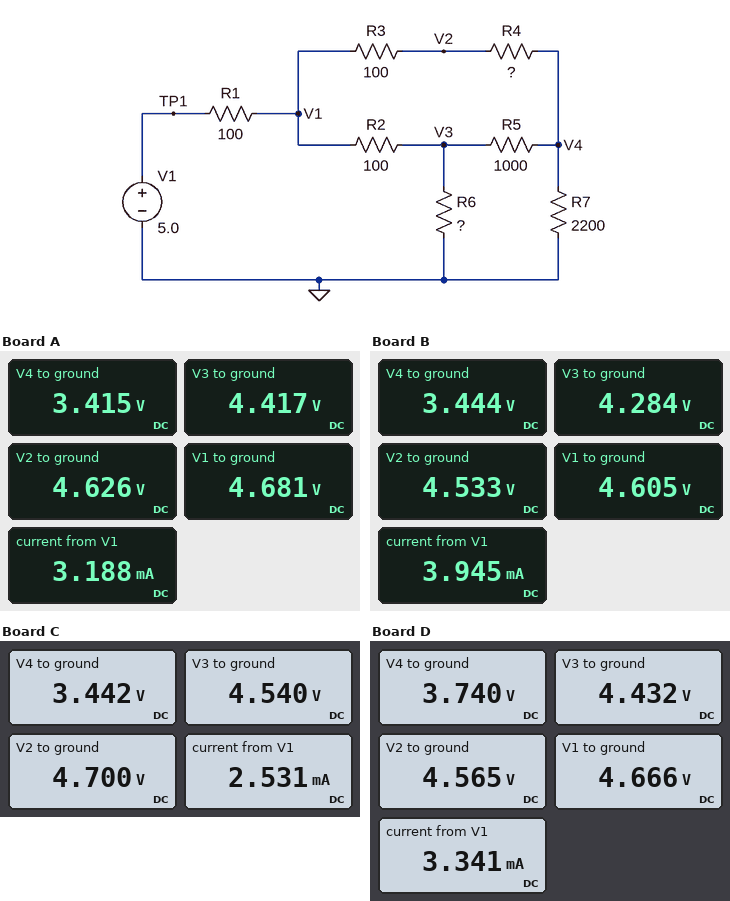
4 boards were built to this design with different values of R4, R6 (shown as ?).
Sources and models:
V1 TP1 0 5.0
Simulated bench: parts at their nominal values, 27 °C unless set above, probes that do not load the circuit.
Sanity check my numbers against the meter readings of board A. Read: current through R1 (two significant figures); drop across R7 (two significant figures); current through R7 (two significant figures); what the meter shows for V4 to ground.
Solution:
3.2 mA
3.4 V
1.6 mA
3.415 V
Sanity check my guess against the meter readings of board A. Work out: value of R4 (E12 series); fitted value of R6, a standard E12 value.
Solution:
2.2 kΩ
2.7 kΩ
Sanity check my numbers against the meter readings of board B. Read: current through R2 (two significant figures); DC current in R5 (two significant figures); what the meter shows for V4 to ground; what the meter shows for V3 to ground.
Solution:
3.2 mA
840 µA
3.444 V
4.284 V
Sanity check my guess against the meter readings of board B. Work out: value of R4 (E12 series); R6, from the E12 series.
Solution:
1.5 kΩ
1.8 kΩ
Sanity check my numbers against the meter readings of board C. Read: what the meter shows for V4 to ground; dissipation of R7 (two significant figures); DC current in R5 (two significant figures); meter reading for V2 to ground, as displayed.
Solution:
3.442 V
5.4 mW
1.1 mA
4.700 V
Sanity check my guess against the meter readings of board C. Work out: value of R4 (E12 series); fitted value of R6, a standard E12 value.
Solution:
2.7 kΩ
4.7 kΩ
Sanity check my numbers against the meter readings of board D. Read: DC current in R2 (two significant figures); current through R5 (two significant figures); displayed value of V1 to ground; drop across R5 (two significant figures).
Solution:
2.3 mA
690 µA
4.666 V
690 mV
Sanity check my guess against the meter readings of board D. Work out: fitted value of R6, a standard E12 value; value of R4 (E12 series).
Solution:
2.7 kΩ
820 Ω
